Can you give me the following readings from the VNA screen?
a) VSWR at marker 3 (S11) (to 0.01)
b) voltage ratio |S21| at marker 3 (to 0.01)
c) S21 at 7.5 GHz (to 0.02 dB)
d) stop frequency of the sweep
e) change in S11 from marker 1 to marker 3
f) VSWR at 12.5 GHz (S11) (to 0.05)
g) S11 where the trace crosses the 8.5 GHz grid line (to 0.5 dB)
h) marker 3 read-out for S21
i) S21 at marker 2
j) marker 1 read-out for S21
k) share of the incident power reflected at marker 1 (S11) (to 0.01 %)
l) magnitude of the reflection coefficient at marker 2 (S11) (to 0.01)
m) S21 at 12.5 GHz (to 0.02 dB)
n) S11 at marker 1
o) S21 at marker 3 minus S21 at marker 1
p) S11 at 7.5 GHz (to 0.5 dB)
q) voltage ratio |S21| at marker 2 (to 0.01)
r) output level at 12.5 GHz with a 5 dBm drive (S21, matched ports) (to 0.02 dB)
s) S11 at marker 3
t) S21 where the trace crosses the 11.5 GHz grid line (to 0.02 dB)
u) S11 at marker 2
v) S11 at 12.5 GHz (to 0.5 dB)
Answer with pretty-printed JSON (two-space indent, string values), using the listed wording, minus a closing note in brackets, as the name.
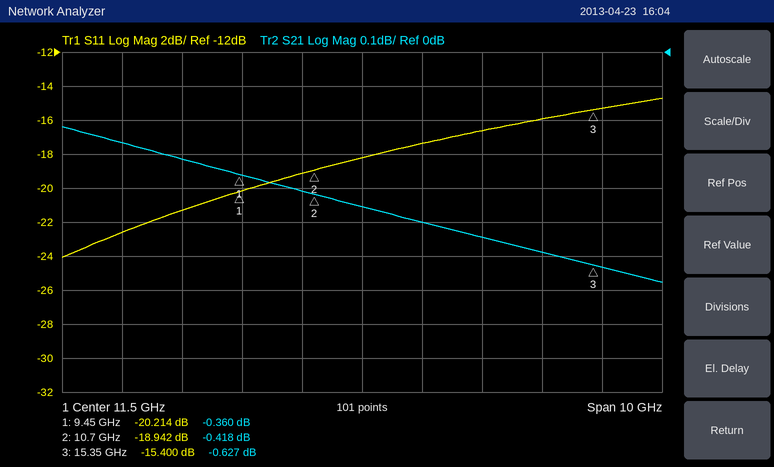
{
  "VSWR at marker 3 (S11)": "1.41",
  "voltage ratio |S21| at marker 3": "0.93",
  "S21 at 7.5 GHz": "-0.26 dB",
  "stop frequency of the sweep": "16.5 GHz",
  "change in S11 from marker 1 to marker 3": "4.814 dB",
  "VSWR at 12.5 GHz (S11)": "1.30",
  "S11 where the trace crosses the 8.5 GHz grid line": "-21.5 dB",
  "marker 3 read-out for S21": "-0.627 dB",
  "S21 at marker 2": "-0.418 dB",
  "marker 1 read-out for S21": "-0.360 dB",
  "share of the incident power reflected at marker 1 (S11)": "0.95 %",
  "magnitude of the reflection coefficient at marker 2 (S11)": "0.11",
  "S21 at 12.5 GHz": "-0.50 dB",
  "S11 at marker 1": "-20.214 dB",
  "S21 at marker 3 minus S21 at marker 1": "-0.267 dB",
  "S11 at 7.5 GHz": "-22.5 dB",
  "voltage ratio |S21| at marker 2": "0.95",
  "output level at 12.5 GHz with a 5 dBm drive (S21, matched ports)": "4.50 dBm",
  "S11 at marker 3": "-15.400 dB",
  "S21 where the trace crosses the 11.5 GHz grid line": "-0.46 dB",
  "S11 at marker 2": "-18.942 dB",
  "S11 at 12.5 GHz": "-17.5 dB"
}
